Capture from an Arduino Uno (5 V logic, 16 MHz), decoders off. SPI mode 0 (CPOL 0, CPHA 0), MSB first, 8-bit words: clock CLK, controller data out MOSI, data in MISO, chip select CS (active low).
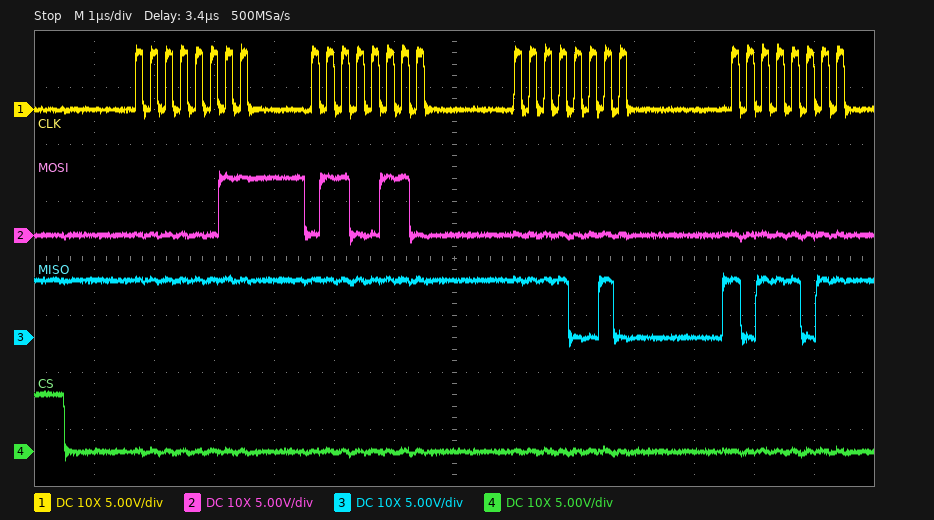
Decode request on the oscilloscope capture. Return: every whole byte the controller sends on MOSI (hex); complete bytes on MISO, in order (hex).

0x03 0x66 0x00 0x00
0xFF 0xFF 0xF2 0xBB
